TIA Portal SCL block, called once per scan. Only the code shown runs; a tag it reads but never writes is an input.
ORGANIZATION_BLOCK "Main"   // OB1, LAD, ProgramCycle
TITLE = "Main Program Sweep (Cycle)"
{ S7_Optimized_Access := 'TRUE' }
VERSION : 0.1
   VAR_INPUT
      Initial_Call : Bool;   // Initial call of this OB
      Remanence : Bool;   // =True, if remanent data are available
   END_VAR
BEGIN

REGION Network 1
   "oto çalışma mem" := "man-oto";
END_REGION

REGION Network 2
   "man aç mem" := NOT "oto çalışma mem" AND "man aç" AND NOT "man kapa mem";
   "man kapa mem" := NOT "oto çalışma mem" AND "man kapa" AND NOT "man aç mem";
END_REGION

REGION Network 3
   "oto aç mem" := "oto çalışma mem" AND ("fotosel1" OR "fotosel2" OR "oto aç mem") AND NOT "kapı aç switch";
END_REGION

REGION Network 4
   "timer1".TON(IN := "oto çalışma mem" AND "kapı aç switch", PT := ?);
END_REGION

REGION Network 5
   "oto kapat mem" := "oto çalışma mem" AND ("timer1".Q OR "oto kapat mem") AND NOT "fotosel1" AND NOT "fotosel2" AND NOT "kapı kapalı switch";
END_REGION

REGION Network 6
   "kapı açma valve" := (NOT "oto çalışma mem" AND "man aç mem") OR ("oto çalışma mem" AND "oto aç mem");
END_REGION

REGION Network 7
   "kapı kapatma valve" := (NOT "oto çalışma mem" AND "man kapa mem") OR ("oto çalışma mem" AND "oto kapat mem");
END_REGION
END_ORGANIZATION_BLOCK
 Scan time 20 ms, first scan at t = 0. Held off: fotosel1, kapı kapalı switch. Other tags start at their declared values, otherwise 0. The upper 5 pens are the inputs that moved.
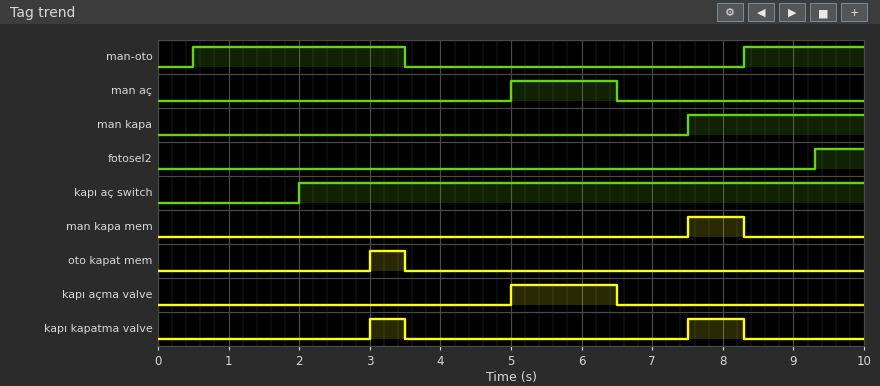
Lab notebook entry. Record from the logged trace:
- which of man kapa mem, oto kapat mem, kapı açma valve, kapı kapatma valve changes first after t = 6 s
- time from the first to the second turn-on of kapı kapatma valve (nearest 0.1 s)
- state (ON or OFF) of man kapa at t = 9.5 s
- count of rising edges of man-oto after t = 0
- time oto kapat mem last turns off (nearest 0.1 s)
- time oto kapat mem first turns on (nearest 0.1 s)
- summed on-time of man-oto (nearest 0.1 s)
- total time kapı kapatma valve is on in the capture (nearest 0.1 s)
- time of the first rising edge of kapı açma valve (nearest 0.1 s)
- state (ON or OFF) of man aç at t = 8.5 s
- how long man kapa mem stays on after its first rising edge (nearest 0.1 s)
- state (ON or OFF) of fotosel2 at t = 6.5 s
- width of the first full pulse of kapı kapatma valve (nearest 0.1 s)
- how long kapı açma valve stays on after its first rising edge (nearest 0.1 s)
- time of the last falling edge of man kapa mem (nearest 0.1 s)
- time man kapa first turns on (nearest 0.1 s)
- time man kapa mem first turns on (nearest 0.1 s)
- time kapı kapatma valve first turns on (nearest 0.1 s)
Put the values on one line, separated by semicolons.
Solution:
kapı açma valve; 4.5 s; ON; 2; 3.5 s; 3.0 s; 4.7 s; 1.3 s; 5.0 s; OFF; 0.8 s; OFF; 0.5 s; 1.5 s; 8.3 s; 7.5 s; 7.5 s; 3.0 s
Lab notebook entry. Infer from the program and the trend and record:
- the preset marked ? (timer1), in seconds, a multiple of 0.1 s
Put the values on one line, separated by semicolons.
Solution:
1.0 s
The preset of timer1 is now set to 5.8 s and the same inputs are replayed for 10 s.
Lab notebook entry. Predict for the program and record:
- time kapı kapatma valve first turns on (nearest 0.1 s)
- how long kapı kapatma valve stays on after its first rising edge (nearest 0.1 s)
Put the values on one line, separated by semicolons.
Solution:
7.5 s; 0.8 s
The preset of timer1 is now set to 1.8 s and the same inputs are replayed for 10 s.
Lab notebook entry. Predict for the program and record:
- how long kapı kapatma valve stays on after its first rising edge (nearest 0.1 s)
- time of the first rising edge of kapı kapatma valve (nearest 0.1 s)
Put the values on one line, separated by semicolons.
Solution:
0.8 s; 7.5 s
